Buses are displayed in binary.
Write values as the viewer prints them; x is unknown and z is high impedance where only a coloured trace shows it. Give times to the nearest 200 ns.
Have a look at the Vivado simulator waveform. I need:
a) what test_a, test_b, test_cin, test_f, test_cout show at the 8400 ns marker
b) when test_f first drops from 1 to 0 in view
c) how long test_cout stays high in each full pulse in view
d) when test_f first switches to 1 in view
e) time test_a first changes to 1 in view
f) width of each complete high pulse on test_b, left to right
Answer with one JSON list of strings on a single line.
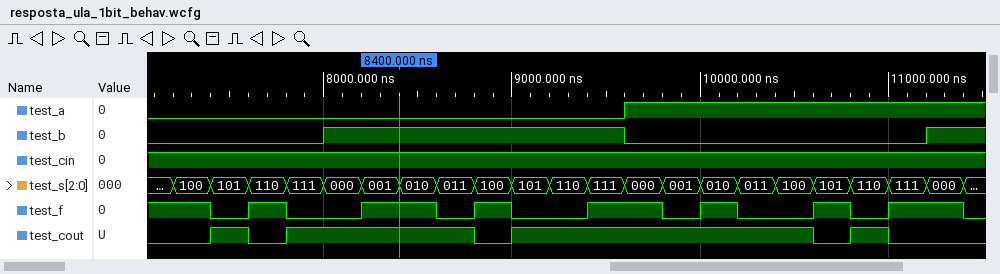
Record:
["test_a=0, test_b=1, test_cin=1, test_f=1, test_cout=1", "7400 ns", "200 ns, 1000 ns, 1600 ns, 200 ns", "7600 ns", "9600 ns", "1600 ns"]
